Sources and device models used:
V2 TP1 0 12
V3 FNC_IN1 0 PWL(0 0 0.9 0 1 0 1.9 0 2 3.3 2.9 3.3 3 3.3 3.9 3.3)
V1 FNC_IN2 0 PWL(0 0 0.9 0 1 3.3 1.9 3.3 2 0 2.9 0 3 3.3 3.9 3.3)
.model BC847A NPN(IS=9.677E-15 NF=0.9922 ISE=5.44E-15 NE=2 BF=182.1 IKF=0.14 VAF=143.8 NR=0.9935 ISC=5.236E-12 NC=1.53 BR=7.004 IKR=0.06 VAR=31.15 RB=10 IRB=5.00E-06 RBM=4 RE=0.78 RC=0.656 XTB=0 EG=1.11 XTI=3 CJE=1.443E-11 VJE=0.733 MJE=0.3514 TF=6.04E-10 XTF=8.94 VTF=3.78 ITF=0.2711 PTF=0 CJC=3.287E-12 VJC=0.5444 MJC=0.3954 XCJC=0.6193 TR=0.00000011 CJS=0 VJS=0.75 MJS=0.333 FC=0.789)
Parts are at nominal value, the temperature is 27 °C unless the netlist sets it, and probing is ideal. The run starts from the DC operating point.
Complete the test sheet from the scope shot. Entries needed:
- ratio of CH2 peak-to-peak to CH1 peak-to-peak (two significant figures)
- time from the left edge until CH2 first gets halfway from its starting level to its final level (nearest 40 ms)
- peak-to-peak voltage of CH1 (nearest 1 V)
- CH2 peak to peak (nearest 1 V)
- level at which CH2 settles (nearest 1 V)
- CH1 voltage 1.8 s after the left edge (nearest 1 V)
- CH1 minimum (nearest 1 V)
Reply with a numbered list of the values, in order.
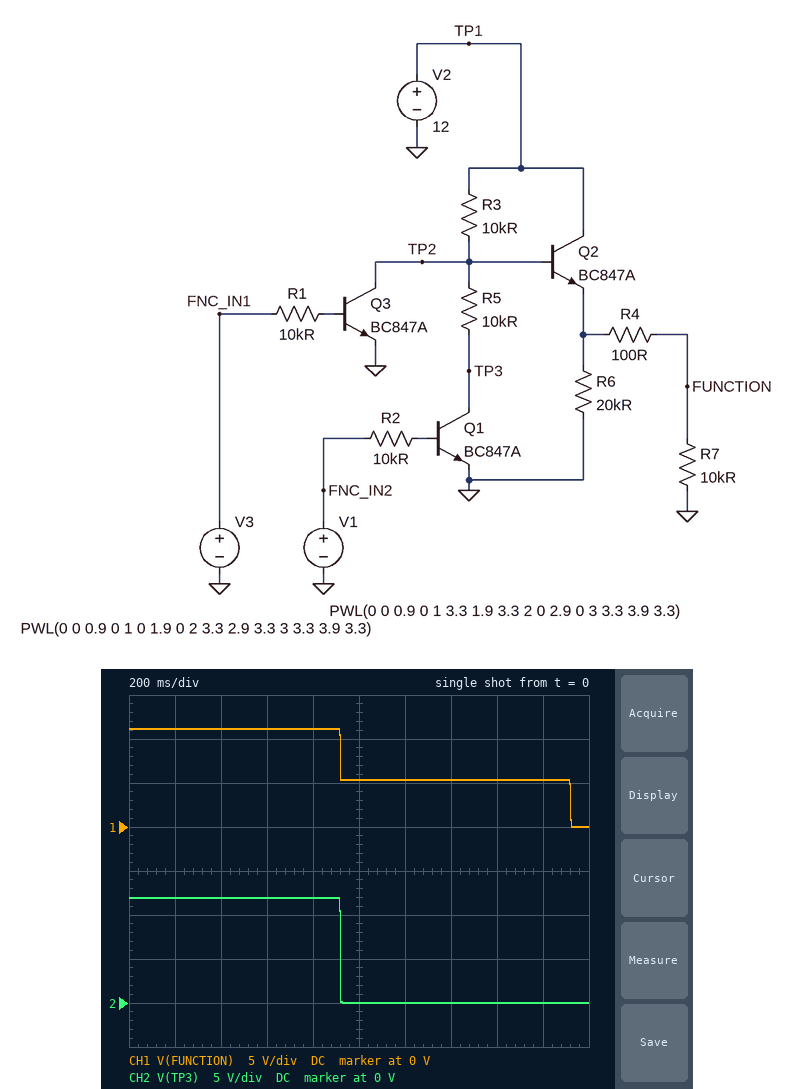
1. 1.1
2. 920 ms
3. 11 V
4. 12 V
5. 0 V
6. 5 V
7. 0 V
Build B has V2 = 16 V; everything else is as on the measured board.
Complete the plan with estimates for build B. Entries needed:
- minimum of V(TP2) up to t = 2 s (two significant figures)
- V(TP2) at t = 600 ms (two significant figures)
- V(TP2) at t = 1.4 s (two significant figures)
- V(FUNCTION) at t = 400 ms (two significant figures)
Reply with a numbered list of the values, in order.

1. 27 mV
2. 16 V
3. 8.0 V
4. 15 V
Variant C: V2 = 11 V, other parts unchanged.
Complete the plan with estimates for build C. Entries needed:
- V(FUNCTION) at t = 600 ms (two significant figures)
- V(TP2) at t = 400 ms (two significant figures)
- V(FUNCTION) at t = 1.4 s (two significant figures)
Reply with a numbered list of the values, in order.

1. 10 V
2. 11 V
3. 4.8 V
